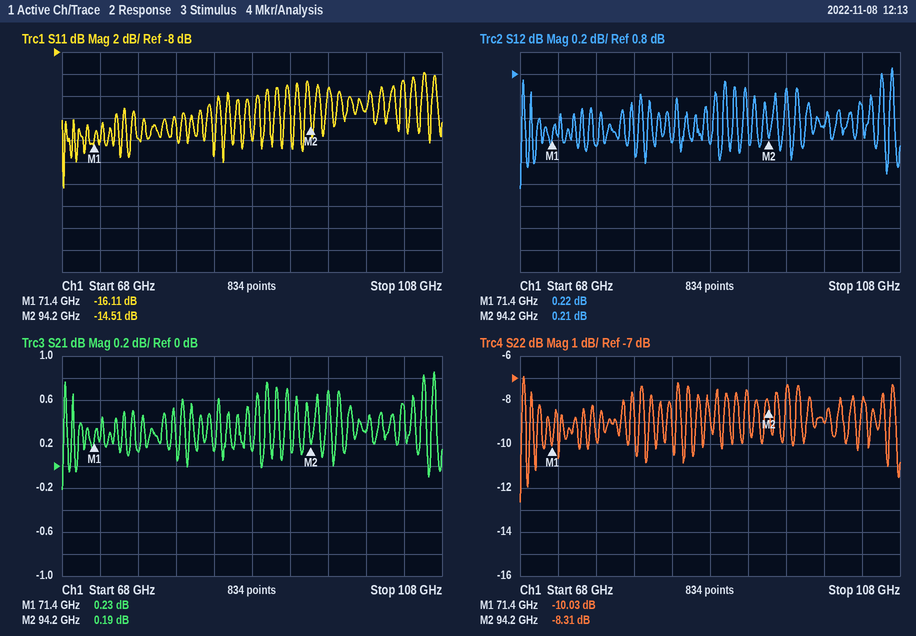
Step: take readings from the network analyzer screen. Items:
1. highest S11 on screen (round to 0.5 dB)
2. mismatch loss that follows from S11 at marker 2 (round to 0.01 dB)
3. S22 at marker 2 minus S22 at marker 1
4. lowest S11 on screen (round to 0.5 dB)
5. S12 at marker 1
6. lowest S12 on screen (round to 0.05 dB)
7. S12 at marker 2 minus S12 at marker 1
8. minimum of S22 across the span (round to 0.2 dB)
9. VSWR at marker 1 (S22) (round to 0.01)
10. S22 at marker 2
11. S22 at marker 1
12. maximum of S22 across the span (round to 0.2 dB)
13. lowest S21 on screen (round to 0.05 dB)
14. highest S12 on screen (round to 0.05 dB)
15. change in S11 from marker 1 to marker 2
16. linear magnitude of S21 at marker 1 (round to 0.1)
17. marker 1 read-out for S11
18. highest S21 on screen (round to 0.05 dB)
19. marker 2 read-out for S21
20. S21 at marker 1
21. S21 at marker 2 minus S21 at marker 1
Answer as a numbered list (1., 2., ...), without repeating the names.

1. -10.0 dB
2. 0.16 dB
3. 1.72 dB
4. -20.5 dB
5. 0.22 dB
6. -0.25 dB
7. -0.01 dB
8. -12.6 dB
9. 1.92
10. -8.31 dB
11. -10.03 dB
12. -7.0 dB
13. -0.20 dB
14. 0.85 dB
15. 1.60 dB
16. 1.0
17. -16.11 dB
18. 0.85 dB
19. 0.19 dB
20. 0.23 dB
21. -0.04 dB
